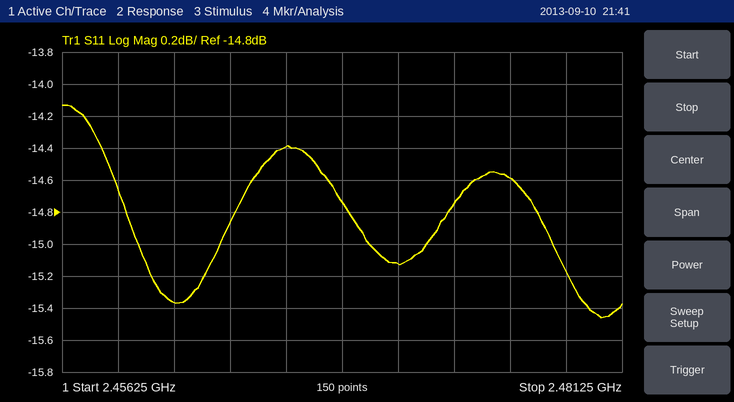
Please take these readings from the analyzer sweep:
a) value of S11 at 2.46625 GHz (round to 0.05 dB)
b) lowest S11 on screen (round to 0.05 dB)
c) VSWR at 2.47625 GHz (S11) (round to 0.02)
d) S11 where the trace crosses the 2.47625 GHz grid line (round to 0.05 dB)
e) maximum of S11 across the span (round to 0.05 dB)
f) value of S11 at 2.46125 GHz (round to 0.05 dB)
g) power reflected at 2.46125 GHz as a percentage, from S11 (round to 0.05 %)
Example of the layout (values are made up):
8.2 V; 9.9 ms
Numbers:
-14.40 dB; -15.45 dB; 1.46; -14.60 dB; -14.15 dB; -15.35 dB; 2.90 %
